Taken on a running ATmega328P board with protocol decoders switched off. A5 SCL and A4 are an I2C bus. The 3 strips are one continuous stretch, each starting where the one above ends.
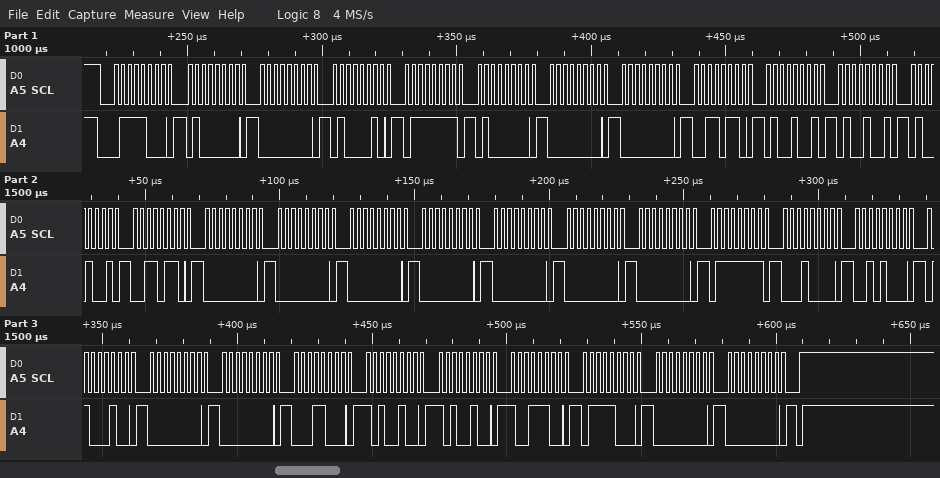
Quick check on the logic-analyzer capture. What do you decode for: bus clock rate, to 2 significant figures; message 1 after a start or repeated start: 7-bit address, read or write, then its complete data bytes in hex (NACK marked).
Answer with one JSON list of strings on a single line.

["400 kHz", "0x3C write: 40 00 42 7F 40 00 00 36 49 49 49 36 00 00 00 00 00 00 00 7F 10 28 44 00 00 18 A4 A4 9C 78 00 00"]
